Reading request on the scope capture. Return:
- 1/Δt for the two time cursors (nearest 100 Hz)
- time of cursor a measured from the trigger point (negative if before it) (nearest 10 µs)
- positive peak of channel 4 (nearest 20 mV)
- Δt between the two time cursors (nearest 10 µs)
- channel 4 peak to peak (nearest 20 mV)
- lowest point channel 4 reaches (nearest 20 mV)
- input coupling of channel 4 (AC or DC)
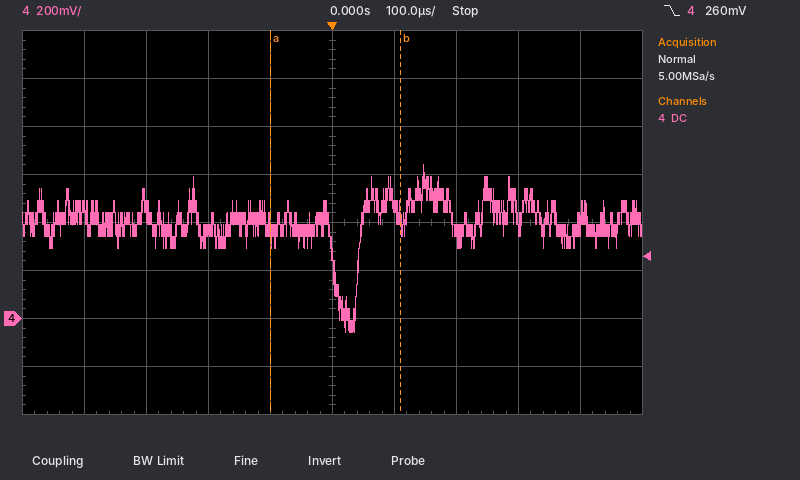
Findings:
4.8 kHz
-100 µs
640 mV
210 µs
700 mV
-60 mV
DC
